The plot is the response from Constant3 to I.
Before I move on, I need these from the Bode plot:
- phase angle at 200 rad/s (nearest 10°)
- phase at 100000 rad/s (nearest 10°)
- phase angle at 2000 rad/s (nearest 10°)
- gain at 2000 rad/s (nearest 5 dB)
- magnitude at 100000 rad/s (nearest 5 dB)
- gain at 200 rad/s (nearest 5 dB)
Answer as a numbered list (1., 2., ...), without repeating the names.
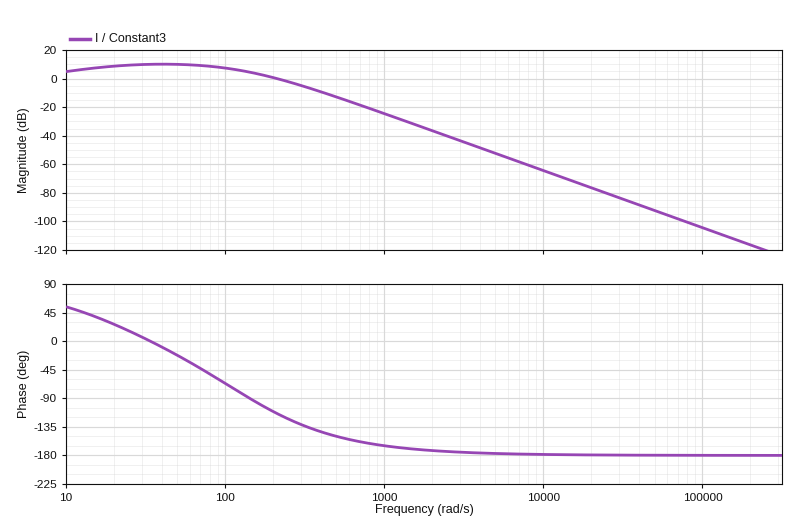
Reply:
1. -110°
2. -180°
3. -170°
4. -35 dB
5. -105 dB
6. 0 dB
